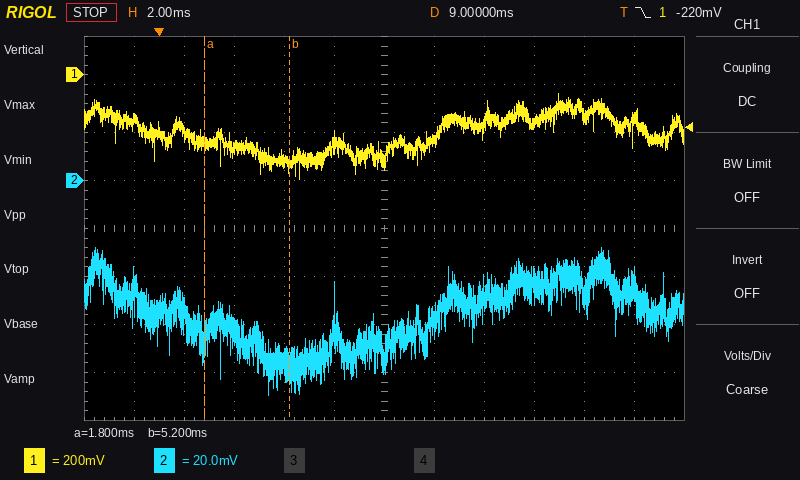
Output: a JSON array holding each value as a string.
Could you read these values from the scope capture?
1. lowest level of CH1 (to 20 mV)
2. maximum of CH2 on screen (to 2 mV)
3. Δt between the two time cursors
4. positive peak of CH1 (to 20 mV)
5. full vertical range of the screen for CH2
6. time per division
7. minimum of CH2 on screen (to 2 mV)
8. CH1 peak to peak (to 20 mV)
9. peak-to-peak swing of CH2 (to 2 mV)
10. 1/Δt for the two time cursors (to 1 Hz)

["-440 mV", "-28 mV", "3.4 ms", "-80 mV", "160 mV", "2 ms", "-90 mV", "360 mV", "62 mV", "294 Hz"]
